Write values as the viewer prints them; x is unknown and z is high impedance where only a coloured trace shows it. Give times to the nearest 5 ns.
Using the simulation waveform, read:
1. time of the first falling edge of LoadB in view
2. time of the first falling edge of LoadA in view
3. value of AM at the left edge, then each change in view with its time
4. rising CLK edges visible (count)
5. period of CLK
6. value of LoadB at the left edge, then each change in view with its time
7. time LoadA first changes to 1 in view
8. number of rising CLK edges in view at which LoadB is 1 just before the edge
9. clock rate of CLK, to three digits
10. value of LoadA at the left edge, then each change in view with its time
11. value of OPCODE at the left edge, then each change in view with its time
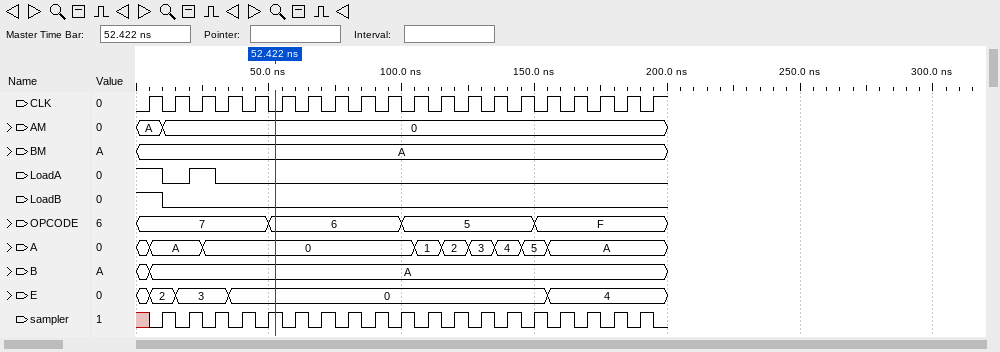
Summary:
10 ns
10 ns
A, 0 at 10 ns
20
10 ns
1, 0 at 10 ns
20 ns
1
100 MHz
1, 0 at 10 ns, 1 at 20 ns, 0 at 30 ns
7, 6 at 50 ns, 5 at 100 ns, F at 150 ns
